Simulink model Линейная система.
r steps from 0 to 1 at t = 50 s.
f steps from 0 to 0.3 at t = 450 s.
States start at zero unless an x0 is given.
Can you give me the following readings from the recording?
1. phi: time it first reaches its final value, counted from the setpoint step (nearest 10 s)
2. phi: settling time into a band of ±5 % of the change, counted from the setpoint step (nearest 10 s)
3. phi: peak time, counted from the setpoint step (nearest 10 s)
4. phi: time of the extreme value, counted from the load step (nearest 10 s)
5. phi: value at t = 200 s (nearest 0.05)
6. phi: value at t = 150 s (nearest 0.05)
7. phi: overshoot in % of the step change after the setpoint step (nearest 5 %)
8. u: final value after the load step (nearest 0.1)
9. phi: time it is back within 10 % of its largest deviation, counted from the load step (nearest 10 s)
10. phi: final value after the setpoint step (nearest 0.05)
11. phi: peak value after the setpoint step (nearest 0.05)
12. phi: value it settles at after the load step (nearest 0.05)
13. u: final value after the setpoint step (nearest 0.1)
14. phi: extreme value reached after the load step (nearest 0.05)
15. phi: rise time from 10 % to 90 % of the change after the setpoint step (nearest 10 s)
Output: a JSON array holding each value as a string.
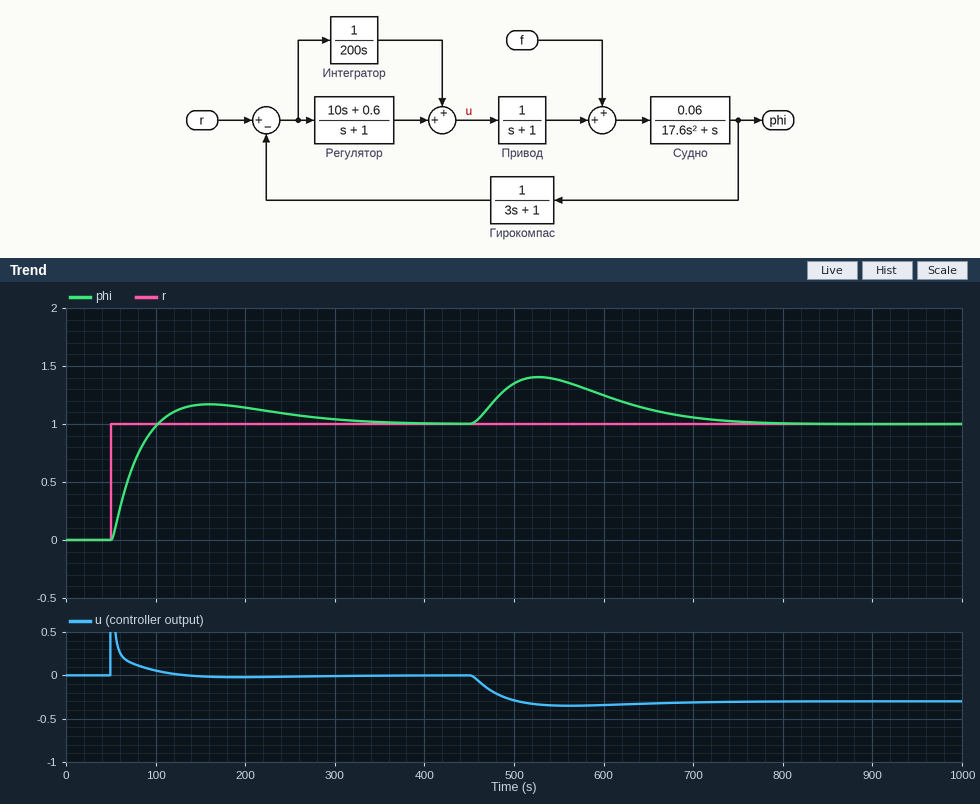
["50 s", "240 s", "110 s", "80 s", "1.15", "1.15", "15 %", "-0.3", "270 s", "1.00", "1.15", "1.00", "0.0", "1.40", "40 s"]
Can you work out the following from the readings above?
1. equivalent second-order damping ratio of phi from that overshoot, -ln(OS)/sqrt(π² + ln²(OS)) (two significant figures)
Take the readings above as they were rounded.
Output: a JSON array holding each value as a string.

["0.52"]
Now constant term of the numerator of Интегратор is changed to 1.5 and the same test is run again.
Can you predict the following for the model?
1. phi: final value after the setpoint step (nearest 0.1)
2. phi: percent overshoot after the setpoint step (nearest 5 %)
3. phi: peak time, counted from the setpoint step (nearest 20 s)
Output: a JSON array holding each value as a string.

["1.0", "25 %", "100 s"]
